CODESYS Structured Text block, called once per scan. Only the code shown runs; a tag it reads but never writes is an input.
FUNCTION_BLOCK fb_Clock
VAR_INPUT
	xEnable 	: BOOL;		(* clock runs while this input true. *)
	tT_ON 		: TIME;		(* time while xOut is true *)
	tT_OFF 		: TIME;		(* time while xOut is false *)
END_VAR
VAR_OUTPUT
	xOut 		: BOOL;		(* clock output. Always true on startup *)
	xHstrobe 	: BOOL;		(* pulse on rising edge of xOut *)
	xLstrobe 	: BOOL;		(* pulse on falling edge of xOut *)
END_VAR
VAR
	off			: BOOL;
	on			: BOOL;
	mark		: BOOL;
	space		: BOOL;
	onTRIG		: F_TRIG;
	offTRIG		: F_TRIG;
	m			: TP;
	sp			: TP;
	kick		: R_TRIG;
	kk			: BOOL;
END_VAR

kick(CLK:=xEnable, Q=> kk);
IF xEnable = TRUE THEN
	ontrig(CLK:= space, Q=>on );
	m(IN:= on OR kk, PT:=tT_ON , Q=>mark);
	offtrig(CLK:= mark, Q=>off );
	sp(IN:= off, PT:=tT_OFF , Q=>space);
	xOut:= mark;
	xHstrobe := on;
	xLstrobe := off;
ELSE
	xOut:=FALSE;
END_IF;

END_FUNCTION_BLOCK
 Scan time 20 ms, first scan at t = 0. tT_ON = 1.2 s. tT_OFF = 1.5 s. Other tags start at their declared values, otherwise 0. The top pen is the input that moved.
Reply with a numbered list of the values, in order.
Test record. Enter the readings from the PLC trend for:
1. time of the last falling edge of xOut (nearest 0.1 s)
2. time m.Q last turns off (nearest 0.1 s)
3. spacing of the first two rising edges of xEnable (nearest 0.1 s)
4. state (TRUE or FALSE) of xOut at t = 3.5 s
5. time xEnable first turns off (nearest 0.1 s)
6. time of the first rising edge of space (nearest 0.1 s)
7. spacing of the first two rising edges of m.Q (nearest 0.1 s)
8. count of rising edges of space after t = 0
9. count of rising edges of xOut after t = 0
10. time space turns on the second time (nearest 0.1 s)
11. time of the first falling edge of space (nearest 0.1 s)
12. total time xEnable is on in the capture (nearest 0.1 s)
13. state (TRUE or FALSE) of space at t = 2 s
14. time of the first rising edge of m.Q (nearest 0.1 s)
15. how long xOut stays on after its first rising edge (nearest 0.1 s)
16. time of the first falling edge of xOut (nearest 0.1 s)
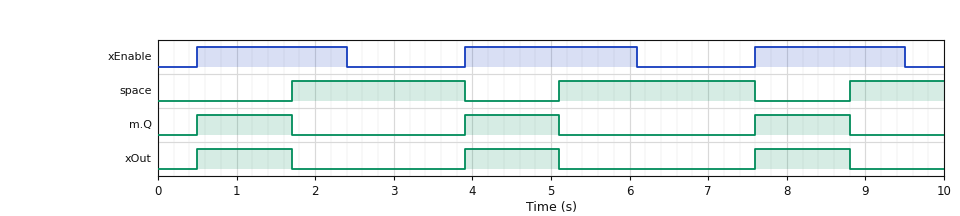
1. 8.8 s
2. 8.8 s
3. 3.4 s
4. FALSE
5. 2.4 s
6. 1.7 s
7. 3.4 s
8. 3
9. 3
10. 5.1 s
11. 3.9 s
12. 6.0 s
13. TRUE
14. 0.5 s
15. 1.2 s
16. 1.7 s
